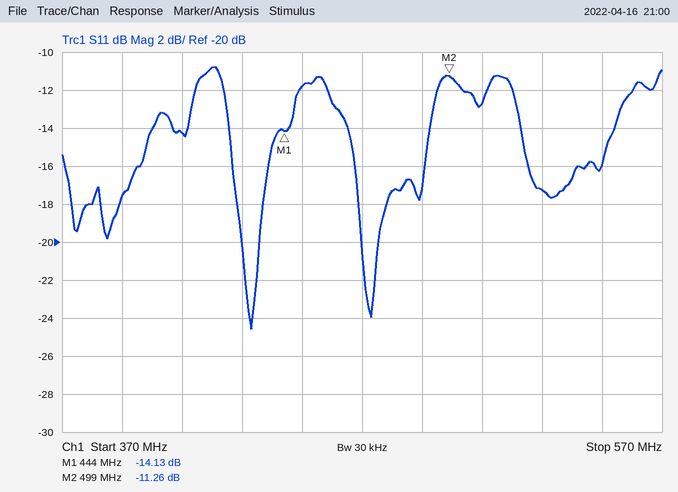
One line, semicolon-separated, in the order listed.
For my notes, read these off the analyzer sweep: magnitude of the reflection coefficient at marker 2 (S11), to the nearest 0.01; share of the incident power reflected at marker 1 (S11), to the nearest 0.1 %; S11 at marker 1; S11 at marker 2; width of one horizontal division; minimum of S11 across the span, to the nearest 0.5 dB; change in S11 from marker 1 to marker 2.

0.27; 3.9 %; -14.13 dB; -11.26 dB; 20 MHz; -24.5 dB; 2.87 dB
